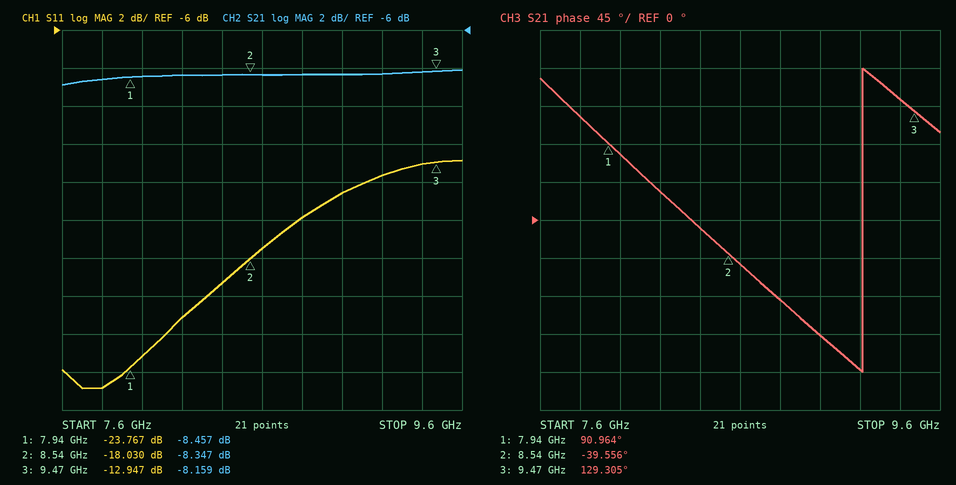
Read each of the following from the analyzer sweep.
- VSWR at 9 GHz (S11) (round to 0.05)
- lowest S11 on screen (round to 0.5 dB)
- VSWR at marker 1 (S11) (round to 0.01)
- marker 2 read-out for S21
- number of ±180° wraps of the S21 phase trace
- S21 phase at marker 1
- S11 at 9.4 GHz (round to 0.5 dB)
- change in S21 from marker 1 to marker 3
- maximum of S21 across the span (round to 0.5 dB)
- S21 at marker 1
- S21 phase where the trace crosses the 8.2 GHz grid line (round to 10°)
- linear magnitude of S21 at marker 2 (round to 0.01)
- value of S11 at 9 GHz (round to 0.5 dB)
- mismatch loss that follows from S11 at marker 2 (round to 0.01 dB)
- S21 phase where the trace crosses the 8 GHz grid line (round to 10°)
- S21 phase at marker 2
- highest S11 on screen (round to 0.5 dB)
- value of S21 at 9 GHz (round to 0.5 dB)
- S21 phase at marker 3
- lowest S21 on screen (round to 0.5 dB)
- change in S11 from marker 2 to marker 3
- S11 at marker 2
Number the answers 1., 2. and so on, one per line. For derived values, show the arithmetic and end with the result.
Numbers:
1. |Γ| = 10^(-14.5/20) = 0.1884; VSWR = (1 + 0.1884)/(1 − 0.1884) ≈ 1.46, so 1.45 to the nearest 0.05
2. -25.0 dB
3. (1 + 0.0648)/(1 − 0.0648) ≈ 1.14
4. -8.347 dB
5. 1
6. 90.964°
7. -13.0 dB
8. -8.159 − (-8.457) = 0.298 dB
9. -8.0 dB
10. -8.457 dB
11. 30°
12. 10^(-8.347/20) ≈ 0.38
13. -14.5 dB
14. −10 log10(1 − 10^(-18.03/10)) ≈ 0.07 dB
15. 80°
16. -39.556°
17. -13.0 dB
18. -8.5 dB
19. 129.305°
20. -9.0 dB
21. -12.947 − (-18.03) = 5.083 dB
22. -18.030 dB
